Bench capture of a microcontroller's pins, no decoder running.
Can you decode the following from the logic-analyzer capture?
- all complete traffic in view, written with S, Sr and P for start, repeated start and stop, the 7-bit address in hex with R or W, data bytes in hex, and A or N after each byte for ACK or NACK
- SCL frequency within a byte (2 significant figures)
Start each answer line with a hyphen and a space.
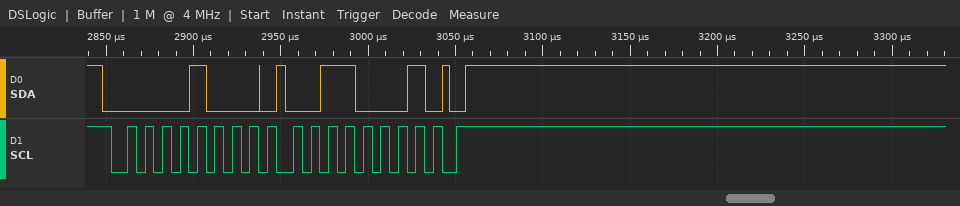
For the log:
- S 04W A 31 A P
- 100 kHz
